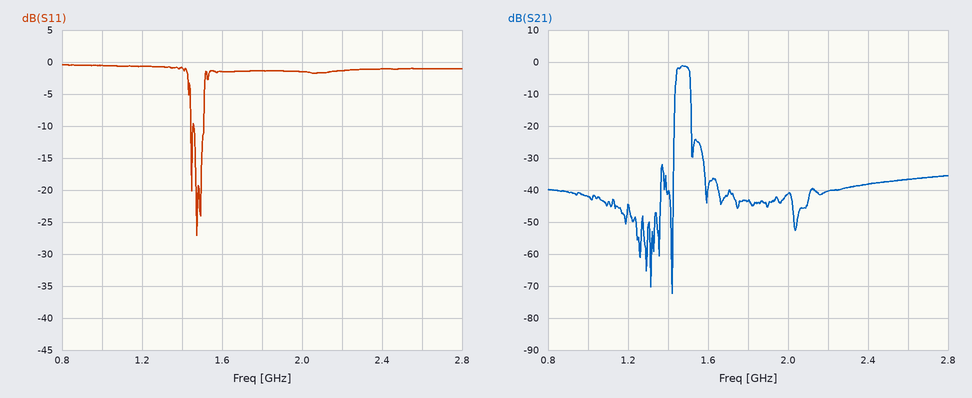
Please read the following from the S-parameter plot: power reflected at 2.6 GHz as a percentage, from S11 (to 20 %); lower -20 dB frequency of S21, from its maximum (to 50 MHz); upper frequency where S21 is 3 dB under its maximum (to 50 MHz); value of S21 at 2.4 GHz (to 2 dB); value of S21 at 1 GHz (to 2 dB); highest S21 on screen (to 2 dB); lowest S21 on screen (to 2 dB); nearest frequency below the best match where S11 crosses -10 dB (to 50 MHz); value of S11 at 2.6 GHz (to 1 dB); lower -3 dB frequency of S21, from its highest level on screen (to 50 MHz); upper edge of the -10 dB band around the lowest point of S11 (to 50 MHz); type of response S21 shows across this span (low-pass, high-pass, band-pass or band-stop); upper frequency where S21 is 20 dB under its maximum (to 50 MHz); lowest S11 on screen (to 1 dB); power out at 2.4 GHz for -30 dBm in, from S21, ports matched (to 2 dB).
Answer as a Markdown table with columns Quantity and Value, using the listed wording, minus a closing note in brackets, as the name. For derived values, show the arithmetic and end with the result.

| Quantity | Value |
|---|---|
| power reflected at 2.6 GHz as a percentage, from S11 | 10^(-1/10) ≈ 79.4 %, so 80 % to the nearest 20 % |
| lower -20 dB frequency of S21, from its maximum | 1.45 GHz |
| upper frequency where S21 is 3 dB under its maximum | 1.50 GHz |
| value of S21 at 2.4 GHz | -38 dB |
| value of S21 at 1 GHz | -42 dB |
| highest S21 on screen | -2 dB |
| lowest S21 on screen | -72 dB |
| nearest frequency below the best match where S11 crosses -10 dB | 1.45 GHz |
| value of S11 at 2.6 GHz | -1 dB |
| lower -3 dB frequency of S21, from its highest level on screen | 1.45 GHz |
| upper edge of the -10 dB band around the lowest point of S11 | 1.50 GHz |
| type of response S21 shows across this span | band-pass |
| upper frequency where S21 is 20 dB under its maximum | 1.50 GHz |
| lowest S11 on screen | -27 dB |
| power out at 2.4 GHz for -30 dBm in, from S21, ports matched | -30 dBm + (-38 dB) = -68 dBm |
